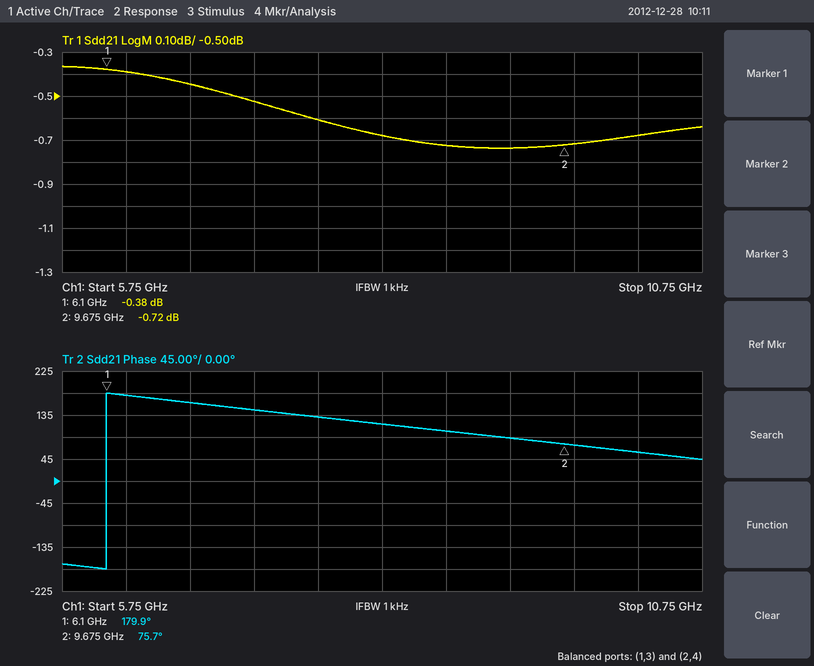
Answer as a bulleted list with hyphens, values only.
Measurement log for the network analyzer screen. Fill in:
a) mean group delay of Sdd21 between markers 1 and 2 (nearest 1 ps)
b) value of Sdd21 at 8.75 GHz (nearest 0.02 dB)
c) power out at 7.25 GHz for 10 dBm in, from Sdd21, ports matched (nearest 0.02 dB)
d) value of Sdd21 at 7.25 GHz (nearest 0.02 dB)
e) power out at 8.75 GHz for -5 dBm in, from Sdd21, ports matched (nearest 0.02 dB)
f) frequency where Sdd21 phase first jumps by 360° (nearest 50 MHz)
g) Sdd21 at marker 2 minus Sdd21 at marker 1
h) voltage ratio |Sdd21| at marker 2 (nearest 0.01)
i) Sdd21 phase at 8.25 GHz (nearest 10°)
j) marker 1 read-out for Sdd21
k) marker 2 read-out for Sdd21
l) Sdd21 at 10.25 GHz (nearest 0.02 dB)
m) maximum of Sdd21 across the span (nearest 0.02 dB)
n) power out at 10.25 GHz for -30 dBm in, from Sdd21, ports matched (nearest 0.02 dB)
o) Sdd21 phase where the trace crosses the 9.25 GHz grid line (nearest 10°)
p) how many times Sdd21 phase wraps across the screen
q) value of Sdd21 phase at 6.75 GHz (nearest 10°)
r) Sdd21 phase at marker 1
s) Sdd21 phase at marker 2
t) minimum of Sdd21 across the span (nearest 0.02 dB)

- 81 ps
- -0.72 dB
- 9.48 dBm
- -0.52 dB
- -5.72 dBm
- 6.10 GHz
- -0.34 dB
- 0.92
- 120°
- -0.38 dB
- -0.72 dB
- -0.68 dB
- -0.36 dB
- -30.68 dBm
- 90°
- 1
- 160°
- 179.9°
- 75.7°
- -0.74 dB
